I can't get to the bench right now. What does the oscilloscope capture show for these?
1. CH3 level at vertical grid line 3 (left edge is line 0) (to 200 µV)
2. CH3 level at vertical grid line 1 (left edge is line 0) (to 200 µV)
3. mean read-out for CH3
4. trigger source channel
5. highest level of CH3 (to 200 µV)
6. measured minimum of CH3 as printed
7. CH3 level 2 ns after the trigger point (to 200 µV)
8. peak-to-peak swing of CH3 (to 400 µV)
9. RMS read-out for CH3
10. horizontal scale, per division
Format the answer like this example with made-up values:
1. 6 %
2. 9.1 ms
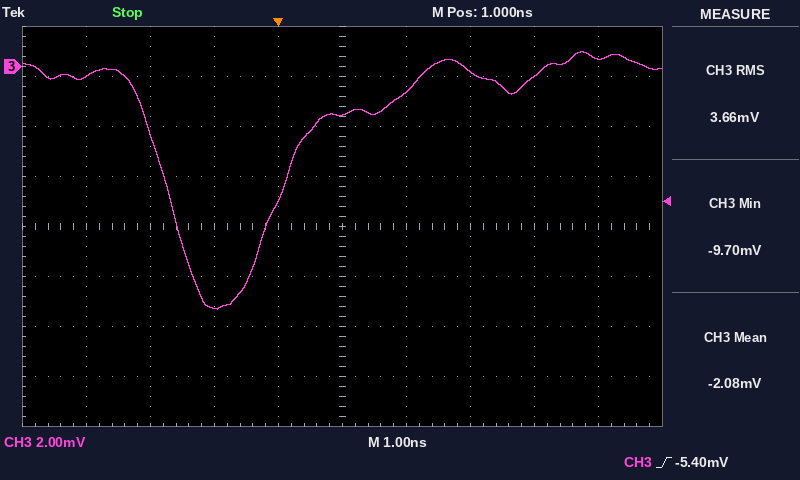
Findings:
1. -9.6 mV
2. -400 µV
3. -2.08 mV
4. CH3
5. 600 µV
6. -9.70 mV
7. -1.0 mV
8. 10.4 mV
9. 3.66 mV
10. 1 ns
